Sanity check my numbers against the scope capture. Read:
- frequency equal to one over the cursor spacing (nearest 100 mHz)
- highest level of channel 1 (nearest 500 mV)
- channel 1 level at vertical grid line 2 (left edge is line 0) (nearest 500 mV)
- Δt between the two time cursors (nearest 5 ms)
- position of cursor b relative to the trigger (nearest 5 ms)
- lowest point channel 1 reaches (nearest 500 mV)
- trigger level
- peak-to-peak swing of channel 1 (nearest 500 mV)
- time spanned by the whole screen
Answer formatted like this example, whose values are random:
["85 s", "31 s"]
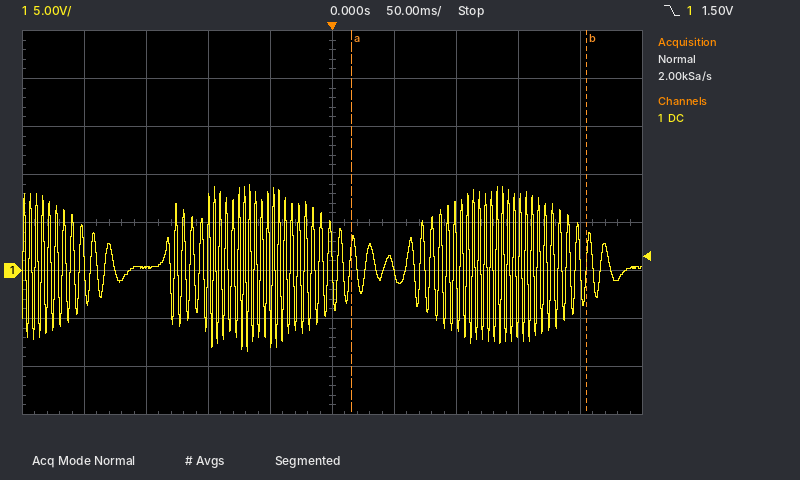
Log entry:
["5.3 Hz", "9.0 V", "500 mV", "190 ms", "+205 ms", "-8.5 V", "1.50 V", "17.5 V", "500 ms"]
